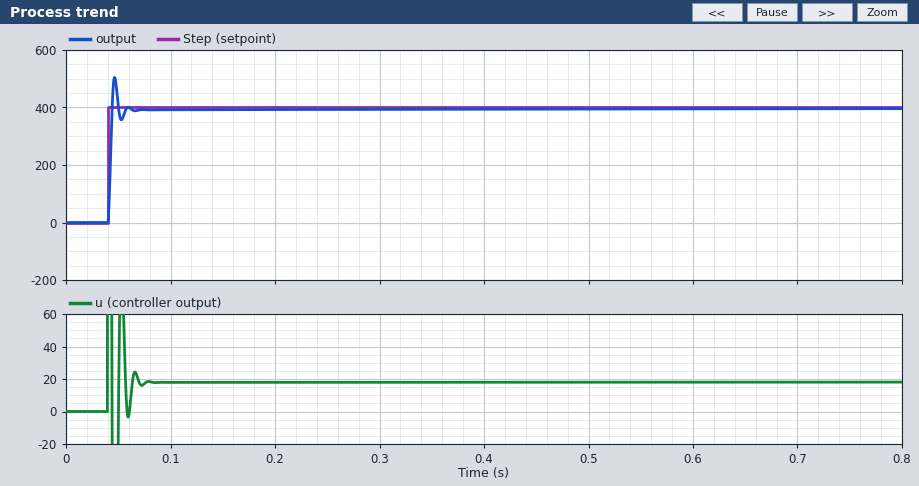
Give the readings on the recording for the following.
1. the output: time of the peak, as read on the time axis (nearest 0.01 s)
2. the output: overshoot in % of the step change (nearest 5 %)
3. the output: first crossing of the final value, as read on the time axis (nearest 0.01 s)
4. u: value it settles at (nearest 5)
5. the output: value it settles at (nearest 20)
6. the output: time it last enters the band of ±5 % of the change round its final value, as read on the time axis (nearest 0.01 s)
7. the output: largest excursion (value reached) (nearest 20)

0.05 s
25 %
0.04 s
20
400
0.06 s
500
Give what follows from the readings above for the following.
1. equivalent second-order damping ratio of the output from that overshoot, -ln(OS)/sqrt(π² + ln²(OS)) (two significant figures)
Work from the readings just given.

0.40
